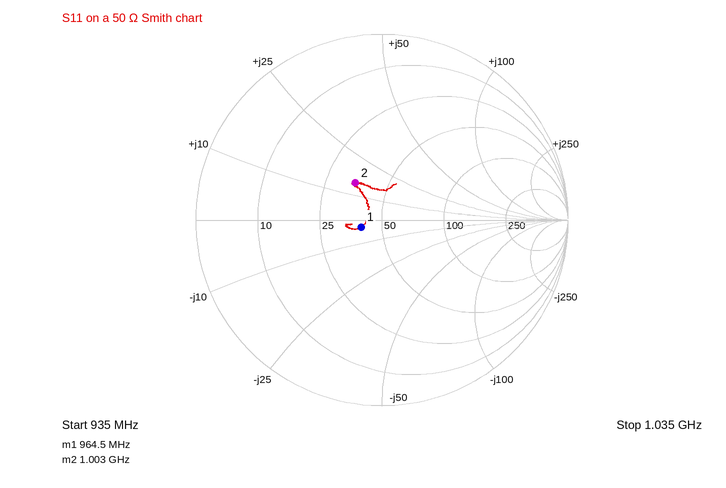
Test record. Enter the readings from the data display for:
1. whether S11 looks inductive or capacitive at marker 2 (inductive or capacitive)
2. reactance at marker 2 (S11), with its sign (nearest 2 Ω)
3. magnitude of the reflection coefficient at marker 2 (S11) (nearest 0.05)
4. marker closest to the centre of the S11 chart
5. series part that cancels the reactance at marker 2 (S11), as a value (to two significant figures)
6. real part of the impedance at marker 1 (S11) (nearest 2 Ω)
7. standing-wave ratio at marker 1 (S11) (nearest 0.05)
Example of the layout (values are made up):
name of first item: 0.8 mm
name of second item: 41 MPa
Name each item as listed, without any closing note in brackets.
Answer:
whether S11 looks inductive or capacitive at marker 2: inductive
reactance at marker 2 (S11), with its sign: +14 Ω
magnitude of the reflection coefficient at marker 2 (S11): 0.25
marker closest to the centre of the S11 chart: marker 1
series part that cancels the reactance at marker 2 (S11), as a value: 11 pF
real part of the impedance at marker 1 (S11): 40 Ω
standing-wave ratio at marker 1 (S11): 1.25
